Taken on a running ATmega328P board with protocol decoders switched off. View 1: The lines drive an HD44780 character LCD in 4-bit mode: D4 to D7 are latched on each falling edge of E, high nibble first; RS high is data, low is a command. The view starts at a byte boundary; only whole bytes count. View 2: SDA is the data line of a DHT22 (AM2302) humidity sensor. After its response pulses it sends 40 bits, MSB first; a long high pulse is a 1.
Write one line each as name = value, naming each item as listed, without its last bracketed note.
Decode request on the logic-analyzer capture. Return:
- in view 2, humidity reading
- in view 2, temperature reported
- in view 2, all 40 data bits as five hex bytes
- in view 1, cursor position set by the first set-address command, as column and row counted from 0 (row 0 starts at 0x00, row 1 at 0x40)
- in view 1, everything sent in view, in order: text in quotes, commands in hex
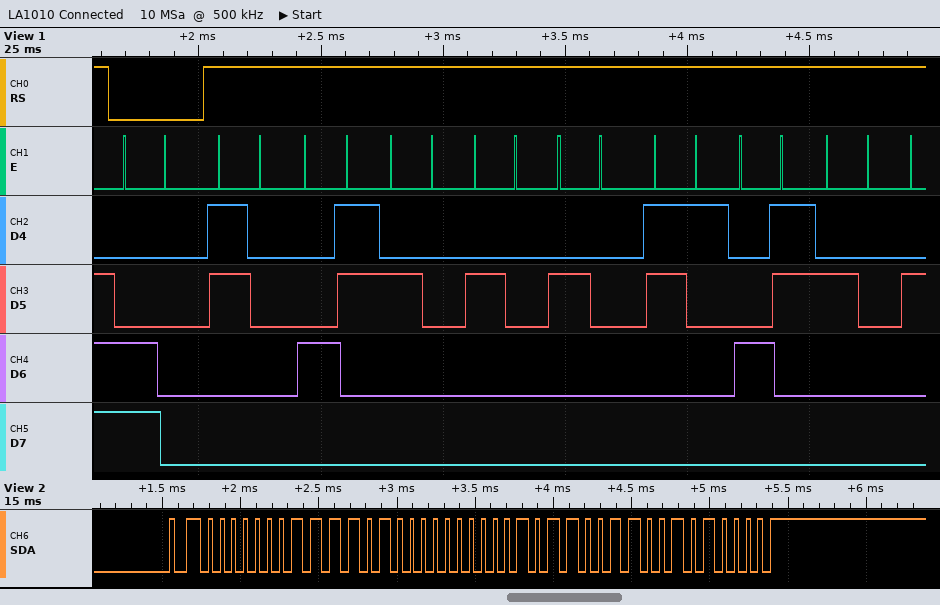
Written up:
in view 2, humidity reading = 48.8 %
in view 2, temperature reported = 35.8 °C
in view 2, all 40 data bits as five hex bytes = 01 E8 01 66 50
in view 1, cursor position set by the first set-address command, as column and row counted from 0 = column 0, row 1
in view 1, everything sent in view, in order: text in quotes, commands in hex = 0xC0 "0C   1C "
